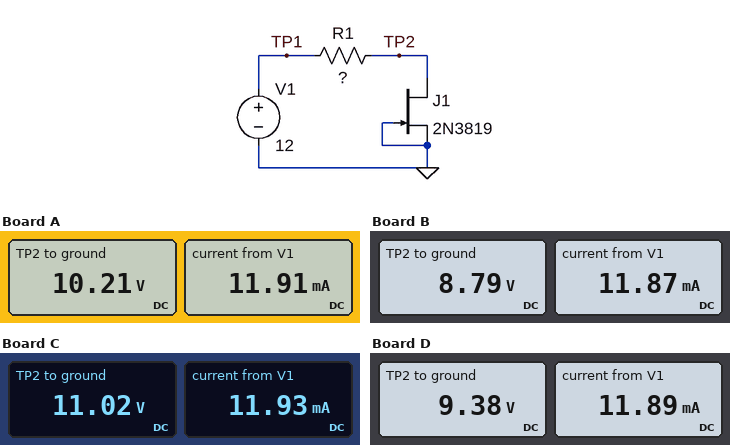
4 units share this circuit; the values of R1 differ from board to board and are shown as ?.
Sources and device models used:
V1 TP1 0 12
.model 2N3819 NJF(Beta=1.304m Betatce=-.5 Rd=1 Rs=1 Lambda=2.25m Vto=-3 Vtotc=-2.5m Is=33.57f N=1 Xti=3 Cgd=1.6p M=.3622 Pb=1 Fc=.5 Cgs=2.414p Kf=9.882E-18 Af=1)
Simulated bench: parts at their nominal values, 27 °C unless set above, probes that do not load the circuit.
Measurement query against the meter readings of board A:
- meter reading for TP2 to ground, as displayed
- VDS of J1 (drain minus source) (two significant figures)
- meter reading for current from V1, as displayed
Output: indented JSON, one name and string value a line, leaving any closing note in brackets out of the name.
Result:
{
  "meter reading for TP2 to ground, as displayed": "10.21 V",
  "VDS of J1 (drain minus source)": "10 V",
  "meter reading for current from V1, as displayed": "11.91 mA"
}
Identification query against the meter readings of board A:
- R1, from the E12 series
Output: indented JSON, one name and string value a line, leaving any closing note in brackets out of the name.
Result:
{
  "R1, from the E12 series": "150 Ω"
}
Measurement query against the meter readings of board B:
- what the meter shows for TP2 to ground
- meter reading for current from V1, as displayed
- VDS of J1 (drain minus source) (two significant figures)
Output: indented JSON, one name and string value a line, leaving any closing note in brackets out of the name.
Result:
{
  "what the meter shows for TP2 to ground": "8.79 V",
  "meter reading for current from V1, as displayed": "11.87 mA",
  "VDS of J1 (drain minus source)": "8.8 V"
}
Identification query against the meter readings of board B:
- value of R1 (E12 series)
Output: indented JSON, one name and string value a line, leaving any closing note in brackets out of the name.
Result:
{
  "value of R1": "270 Ω"
}
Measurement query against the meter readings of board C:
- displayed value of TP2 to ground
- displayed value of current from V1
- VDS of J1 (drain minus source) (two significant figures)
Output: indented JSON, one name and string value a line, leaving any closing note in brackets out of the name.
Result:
{
  "displayed value of TP2 to ground": "11.02 V",
  "displayed value of current from V1": "11.93 mA",
  "VDS of J1 (drain minus source)": "11 V"
}
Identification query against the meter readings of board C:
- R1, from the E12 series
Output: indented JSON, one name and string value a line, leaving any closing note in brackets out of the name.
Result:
{
  "R1, from the E12 series": "82 Ω"
}
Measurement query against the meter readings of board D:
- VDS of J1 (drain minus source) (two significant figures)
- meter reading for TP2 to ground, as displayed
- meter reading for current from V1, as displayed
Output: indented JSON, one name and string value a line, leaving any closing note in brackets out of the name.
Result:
{
  "VDS of J1 (drain minus source)": "9.4 V",
  "meter reading for TP2 to ground, as displayed": "9.38 V",
  "meter reading for current from V1, as displayed": "11.89 mA"
}
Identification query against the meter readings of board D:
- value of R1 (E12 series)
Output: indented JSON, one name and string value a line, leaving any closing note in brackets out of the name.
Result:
{
  "value of R1": "220 Ω"
}
